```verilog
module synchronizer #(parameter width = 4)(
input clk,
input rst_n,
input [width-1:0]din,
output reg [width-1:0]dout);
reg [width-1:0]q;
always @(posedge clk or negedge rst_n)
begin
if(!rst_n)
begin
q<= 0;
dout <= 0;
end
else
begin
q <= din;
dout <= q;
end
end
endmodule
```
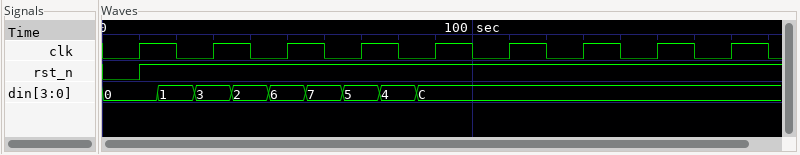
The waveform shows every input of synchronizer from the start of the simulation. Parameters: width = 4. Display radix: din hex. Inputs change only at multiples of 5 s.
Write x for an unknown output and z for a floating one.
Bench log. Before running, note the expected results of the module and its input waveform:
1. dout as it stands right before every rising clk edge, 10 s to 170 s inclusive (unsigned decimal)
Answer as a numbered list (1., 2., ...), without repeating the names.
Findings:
1. 0, 0, 0, 3, 6, 5, 12, 12, 12
